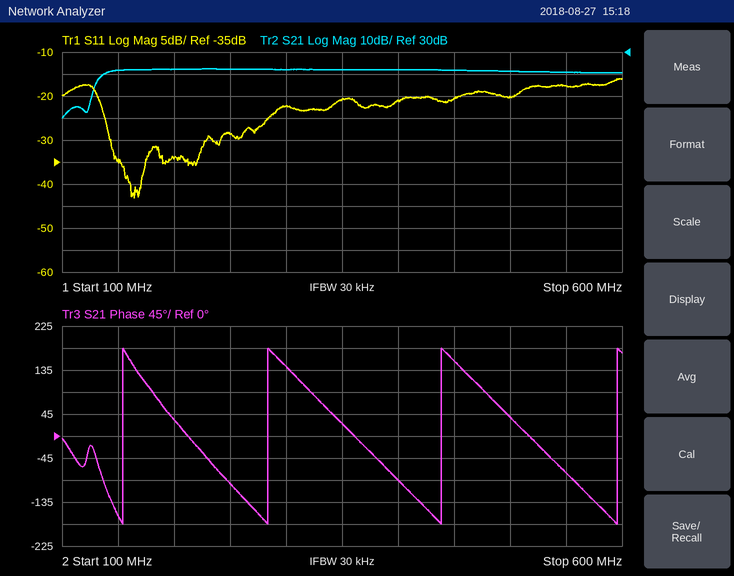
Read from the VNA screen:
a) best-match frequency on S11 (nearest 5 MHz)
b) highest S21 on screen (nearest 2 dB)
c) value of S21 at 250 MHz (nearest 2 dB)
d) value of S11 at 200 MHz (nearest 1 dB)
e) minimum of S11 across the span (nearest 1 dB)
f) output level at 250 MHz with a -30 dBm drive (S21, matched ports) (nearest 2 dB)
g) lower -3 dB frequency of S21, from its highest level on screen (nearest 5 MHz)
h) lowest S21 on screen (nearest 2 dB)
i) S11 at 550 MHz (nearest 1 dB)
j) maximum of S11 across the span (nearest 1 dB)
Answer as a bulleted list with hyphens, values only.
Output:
- 165 MHz
- 22 dB
- 22 dB
- -34 dB
- -43 dB
- -8 dBm
- 135 MHz
- 0 dB
- -18 dB
- -16 dB
